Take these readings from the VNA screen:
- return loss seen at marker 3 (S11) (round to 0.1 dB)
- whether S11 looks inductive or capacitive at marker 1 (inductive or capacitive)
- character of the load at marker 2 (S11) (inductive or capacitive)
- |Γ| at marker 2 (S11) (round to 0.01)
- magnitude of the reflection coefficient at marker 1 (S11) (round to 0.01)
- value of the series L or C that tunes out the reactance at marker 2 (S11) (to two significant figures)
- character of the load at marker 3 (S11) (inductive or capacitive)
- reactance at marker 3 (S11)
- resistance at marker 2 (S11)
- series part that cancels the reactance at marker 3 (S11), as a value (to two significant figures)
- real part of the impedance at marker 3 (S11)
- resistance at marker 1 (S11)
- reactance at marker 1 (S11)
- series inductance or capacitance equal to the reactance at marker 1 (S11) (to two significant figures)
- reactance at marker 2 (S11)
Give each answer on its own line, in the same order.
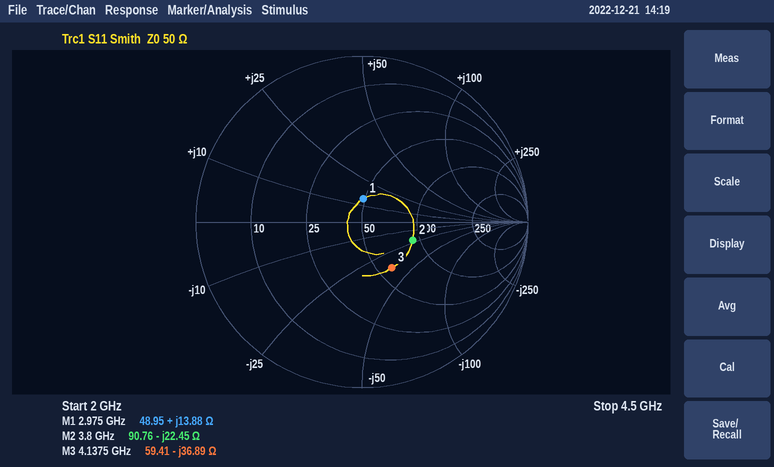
9.6 dB
inductive
capacitive
0.33
0.14
940 pH
capacitive
-36.89 Ω
90.76 Ω
1.4 nH
59.41 Ω
48.95 Ω
+13.88 Ω
740 pH
-22.45 Ω
